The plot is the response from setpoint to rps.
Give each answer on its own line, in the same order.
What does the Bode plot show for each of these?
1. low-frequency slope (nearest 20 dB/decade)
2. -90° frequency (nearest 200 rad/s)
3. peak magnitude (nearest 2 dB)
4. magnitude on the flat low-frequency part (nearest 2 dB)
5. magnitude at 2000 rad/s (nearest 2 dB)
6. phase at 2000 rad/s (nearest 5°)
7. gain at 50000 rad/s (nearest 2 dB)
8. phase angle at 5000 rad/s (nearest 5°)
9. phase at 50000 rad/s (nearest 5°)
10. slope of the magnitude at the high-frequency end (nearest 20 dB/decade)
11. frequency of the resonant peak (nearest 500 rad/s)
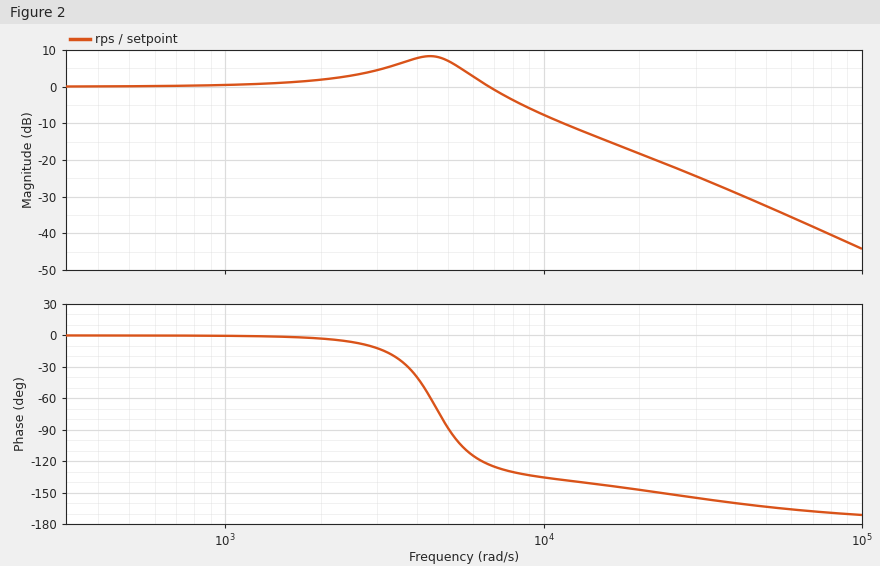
0 dB/decade
5000 rad/s
8 dB
0 dB
2 dB
-5°
-32 dB
-90°
-165°
-40 dB/decade
4500 rad/s
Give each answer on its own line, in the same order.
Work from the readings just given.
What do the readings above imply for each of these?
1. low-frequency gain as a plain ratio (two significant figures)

1.0
